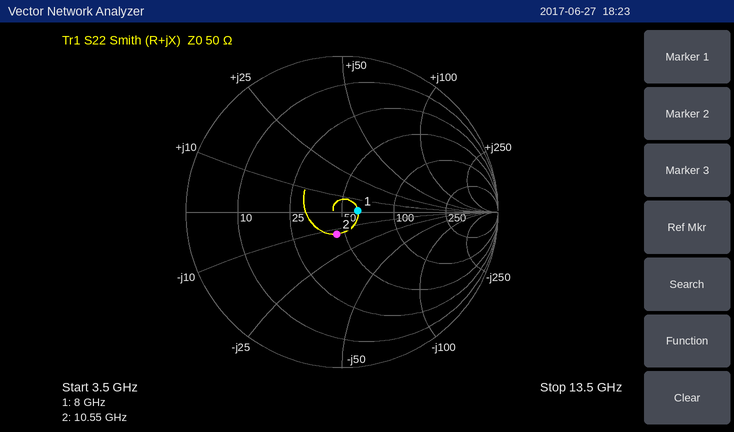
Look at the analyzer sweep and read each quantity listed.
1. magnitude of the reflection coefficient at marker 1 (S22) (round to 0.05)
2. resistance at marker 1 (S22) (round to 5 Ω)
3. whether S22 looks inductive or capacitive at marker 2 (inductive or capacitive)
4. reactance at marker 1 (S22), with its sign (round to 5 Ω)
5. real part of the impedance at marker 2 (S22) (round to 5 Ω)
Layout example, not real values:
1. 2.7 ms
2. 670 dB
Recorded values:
1. 0.10
2. 60 Ω
3. capacitive
4. 0 Ω
5. 45 Ω
